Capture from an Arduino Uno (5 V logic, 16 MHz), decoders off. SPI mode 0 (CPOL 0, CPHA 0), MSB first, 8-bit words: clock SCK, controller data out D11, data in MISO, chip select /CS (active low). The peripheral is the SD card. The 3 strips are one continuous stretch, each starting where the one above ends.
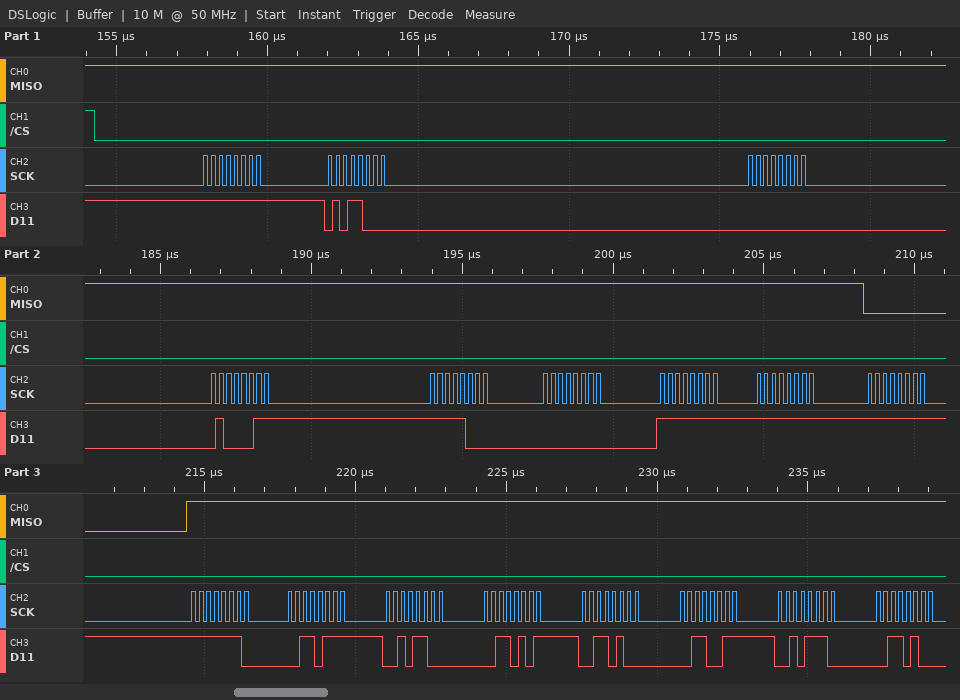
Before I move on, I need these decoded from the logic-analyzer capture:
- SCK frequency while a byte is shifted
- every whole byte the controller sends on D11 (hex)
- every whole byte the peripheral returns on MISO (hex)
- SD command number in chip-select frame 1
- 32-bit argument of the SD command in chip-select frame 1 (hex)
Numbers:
4 MHz
FF 58 00 43 F8 00 FF FF FF FE 37 2C 35 34 33 2E 34
FF FF FF FF FF FF FF FF 00 FF FF FF FF FF FF FF FF
CMD24
0x0043F800
